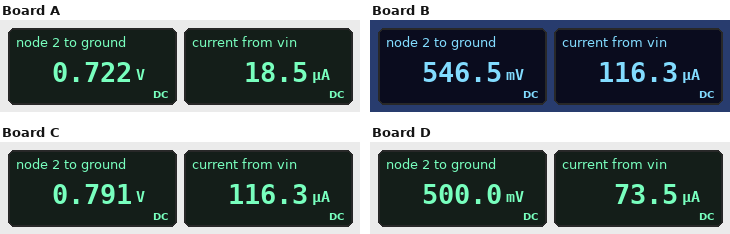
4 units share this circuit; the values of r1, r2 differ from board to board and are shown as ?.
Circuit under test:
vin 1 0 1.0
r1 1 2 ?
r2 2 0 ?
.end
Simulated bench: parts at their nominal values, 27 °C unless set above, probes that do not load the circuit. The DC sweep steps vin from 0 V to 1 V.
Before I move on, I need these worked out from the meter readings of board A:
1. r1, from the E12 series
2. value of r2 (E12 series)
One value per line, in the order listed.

15 kΩ
39 kΩ
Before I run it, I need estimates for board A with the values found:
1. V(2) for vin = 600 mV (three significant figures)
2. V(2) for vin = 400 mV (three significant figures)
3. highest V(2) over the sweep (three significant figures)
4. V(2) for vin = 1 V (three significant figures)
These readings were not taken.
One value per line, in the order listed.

433 mV
289 mV
722 mV
722 mV
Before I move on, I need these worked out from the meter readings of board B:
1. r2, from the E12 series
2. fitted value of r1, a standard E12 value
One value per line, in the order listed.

4.7 kΩ
3.9 kΩ
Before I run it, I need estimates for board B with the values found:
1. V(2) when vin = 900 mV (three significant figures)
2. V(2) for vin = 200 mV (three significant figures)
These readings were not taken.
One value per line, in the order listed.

492 mV
109 mV
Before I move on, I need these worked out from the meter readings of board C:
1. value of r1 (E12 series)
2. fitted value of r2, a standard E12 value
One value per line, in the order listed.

1.8 kΩ
6.8 kΩ
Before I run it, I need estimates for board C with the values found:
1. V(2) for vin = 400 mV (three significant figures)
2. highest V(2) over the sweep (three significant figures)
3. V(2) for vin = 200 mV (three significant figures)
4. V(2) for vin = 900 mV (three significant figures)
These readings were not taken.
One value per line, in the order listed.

316 mV
791 mV
158 mV
712 mV
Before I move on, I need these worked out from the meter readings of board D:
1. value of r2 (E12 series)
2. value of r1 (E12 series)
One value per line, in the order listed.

6.8 kΩ
6.8 kΩ
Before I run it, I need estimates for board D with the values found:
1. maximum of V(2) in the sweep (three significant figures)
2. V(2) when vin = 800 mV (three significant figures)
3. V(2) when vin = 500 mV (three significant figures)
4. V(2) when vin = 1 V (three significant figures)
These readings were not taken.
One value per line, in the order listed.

500 mV
400 mV
250 mV
500 mV
